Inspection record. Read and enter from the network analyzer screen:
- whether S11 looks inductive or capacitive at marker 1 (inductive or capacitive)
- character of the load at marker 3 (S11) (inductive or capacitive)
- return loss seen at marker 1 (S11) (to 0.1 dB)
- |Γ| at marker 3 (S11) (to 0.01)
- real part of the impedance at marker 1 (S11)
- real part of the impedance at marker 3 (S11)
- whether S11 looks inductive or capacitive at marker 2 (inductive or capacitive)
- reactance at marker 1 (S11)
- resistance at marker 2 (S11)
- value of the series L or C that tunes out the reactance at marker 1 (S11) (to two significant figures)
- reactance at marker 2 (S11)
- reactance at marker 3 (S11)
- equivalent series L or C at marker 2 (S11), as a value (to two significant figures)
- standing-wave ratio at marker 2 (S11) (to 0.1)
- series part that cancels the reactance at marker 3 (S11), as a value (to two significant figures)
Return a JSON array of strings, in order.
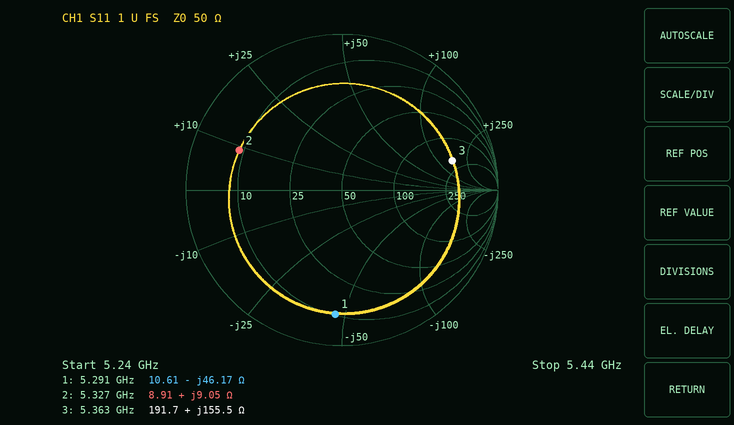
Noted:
["capacitive", "inductive", "2.0 dB", "0.73", "10.61 Ω", "191.7 Ω", "inductive", "-46.17 Ω", "8.91 Ω", "1.4 nH", "+9.05 Ω", "+155.5 Ω", "270 pH", "5.8", "190 fF"]
